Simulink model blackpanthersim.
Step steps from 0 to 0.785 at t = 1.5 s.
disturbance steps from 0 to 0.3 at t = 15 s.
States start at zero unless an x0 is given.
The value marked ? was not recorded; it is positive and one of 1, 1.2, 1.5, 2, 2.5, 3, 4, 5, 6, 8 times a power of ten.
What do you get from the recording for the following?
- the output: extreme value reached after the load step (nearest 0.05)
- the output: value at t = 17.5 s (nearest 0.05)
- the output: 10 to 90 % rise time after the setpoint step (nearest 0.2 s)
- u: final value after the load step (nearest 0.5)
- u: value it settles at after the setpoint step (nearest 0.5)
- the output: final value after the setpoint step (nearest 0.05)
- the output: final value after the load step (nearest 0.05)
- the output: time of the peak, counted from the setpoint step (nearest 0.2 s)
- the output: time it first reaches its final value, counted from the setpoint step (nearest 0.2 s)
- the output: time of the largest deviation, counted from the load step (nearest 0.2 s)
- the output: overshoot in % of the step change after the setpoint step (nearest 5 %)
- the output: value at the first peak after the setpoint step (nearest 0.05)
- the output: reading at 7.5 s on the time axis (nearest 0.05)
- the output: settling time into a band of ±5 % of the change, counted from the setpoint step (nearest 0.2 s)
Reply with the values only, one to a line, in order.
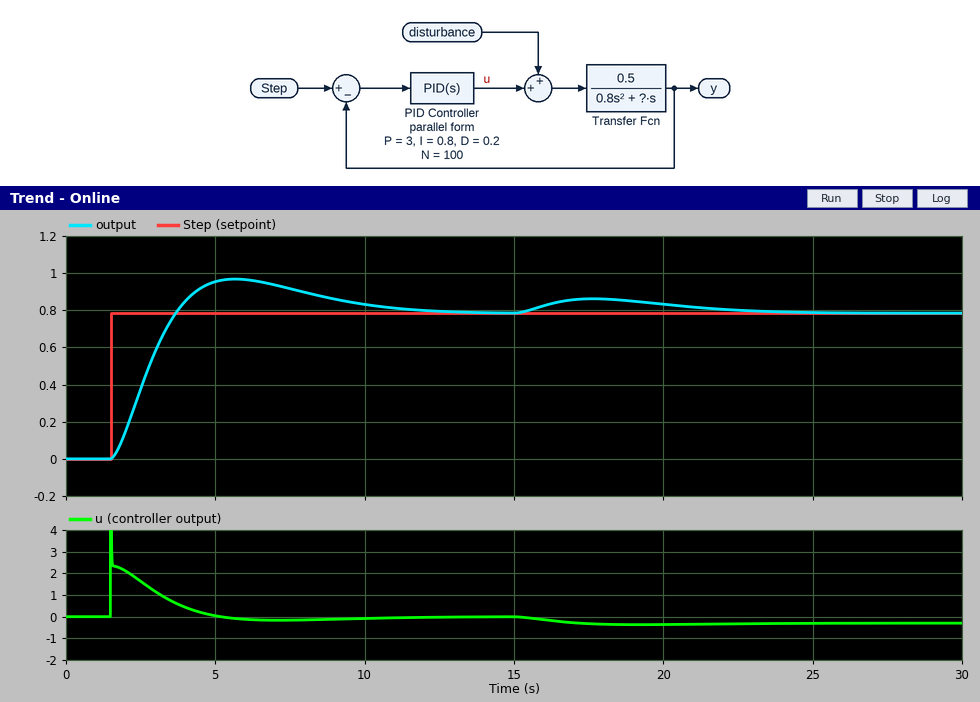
0.85
0.85
1.6 s
-0.5
0.0
0.80
0.80
4.2 s
2.2 s
2.6 s
25 %
0.95
0.90
8.8 s
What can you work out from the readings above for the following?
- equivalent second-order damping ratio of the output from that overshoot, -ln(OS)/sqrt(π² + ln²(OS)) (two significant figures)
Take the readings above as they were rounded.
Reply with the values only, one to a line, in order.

0.40
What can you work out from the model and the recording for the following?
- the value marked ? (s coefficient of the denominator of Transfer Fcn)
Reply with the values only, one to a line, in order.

2
